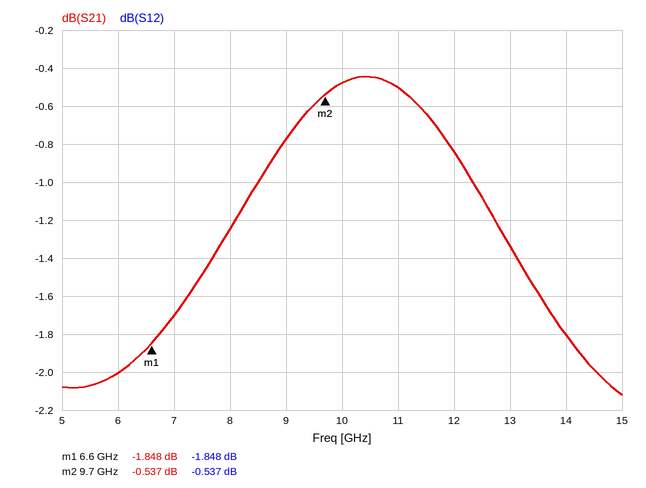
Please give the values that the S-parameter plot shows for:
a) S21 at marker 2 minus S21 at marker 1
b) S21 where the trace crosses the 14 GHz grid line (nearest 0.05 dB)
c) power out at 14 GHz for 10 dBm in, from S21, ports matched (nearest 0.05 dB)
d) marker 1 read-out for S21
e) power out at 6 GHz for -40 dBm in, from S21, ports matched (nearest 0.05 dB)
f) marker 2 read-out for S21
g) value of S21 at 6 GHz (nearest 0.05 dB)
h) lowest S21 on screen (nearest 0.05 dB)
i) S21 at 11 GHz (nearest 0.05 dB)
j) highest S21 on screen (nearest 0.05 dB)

1.311 dB
-1.80 dB
8.20 dBm
-1.848 dB
-42.00 dBm
-0.537 dB
-2.00 dB
-2.10 dB
-0.50 dB
-0.45 dB
